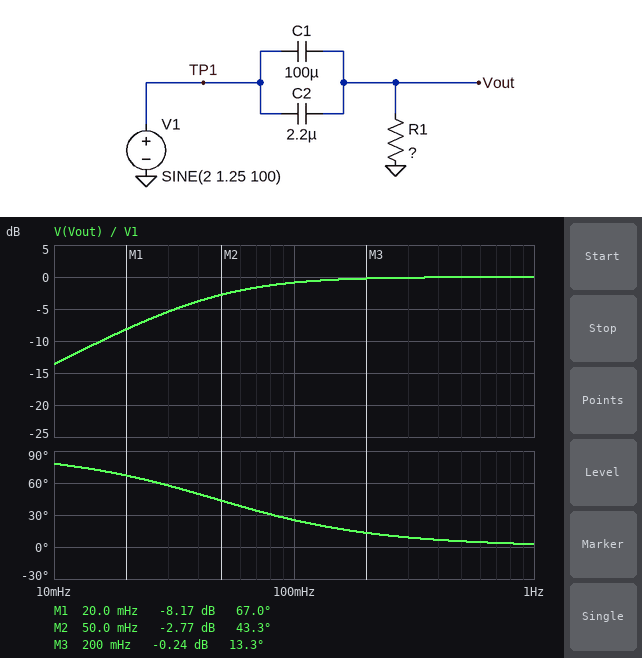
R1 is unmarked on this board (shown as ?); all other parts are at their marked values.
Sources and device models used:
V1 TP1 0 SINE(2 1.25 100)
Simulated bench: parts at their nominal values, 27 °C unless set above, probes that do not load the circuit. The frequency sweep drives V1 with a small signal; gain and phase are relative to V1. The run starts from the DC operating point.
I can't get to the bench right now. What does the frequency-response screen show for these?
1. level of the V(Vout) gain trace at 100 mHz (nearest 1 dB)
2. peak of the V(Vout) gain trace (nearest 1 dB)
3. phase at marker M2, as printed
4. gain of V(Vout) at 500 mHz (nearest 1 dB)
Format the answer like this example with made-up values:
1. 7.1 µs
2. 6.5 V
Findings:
1. -1 dB
2. 0 dB
3. 43.3 deg
4. 0 dB
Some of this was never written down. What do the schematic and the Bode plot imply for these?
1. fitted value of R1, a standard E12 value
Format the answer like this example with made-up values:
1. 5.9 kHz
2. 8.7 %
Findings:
1. 33 kΩ
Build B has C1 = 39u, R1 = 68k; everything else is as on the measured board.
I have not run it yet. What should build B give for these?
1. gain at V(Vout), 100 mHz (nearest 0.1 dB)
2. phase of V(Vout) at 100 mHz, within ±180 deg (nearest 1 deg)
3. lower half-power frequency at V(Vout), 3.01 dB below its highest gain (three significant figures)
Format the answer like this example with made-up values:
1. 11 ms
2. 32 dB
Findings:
1. -1.2 dB
2. 30 deg
3. 56.8 mHz
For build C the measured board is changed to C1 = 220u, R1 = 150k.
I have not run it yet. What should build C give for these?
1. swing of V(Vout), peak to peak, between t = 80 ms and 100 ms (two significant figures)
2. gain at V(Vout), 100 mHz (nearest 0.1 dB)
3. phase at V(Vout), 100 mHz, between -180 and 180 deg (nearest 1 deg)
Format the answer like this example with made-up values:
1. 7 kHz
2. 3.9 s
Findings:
1. 2.5 V
2. 0 dB
3. 3 deg
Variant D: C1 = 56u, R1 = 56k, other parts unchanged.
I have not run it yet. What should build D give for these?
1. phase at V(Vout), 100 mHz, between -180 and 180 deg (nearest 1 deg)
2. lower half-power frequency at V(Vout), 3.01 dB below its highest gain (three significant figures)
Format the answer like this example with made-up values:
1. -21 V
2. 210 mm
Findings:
1. 26 deg
2. 48.8 mHz
